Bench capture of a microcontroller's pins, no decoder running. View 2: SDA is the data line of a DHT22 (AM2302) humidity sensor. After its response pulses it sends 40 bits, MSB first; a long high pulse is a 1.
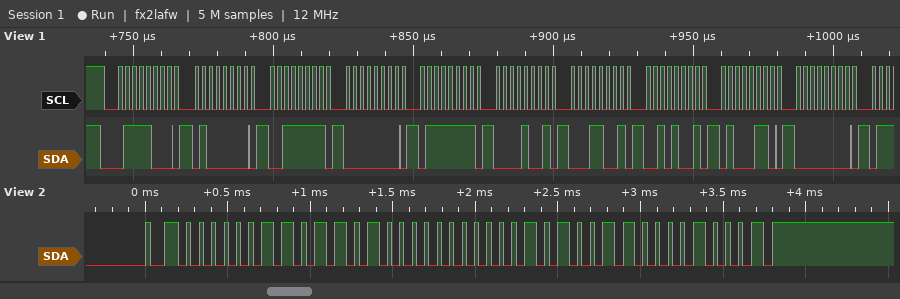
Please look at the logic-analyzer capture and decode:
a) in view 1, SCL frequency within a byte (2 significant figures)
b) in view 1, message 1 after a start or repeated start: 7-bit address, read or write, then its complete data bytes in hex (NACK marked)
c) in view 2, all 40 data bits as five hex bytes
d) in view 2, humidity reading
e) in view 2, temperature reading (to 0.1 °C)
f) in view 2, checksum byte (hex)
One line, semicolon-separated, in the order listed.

400 kHz; 0x3C write: 40 3F 00 7F 09 19 29 46 00; 03 68 00 A6 11; 87.2 %; 16.6 °C; 0x11
